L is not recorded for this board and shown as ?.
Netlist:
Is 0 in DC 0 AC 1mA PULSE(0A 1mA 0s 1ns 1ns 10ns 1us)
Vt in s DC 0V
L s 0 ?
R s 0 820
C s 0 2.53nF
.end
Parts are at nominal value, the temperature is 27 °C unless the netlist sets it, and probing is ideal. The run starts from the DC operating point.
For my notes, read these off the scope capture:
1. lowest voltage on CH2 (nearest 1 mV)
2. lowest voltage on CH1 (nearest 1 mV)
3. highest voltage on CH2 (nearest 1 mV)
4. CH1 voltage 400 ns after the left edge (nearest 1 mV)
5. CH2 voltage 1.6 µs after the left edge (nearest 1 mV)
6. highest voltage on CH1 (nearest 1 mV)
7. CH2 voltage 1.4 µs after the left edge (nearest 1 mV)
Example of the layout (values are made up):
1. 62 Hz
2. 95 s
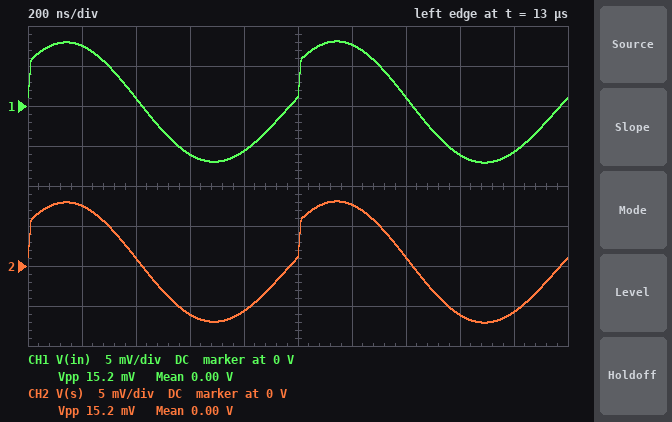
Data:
1. -7 mV
2. -7 mV
3. 8 mV
4. 1 mV
5. -6 mV
6. 8 mV
7. 1 mV
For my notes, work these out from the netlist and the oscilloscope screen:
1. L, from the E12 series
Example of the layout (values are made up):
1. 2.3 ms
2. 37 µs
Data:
1. 12 µH
